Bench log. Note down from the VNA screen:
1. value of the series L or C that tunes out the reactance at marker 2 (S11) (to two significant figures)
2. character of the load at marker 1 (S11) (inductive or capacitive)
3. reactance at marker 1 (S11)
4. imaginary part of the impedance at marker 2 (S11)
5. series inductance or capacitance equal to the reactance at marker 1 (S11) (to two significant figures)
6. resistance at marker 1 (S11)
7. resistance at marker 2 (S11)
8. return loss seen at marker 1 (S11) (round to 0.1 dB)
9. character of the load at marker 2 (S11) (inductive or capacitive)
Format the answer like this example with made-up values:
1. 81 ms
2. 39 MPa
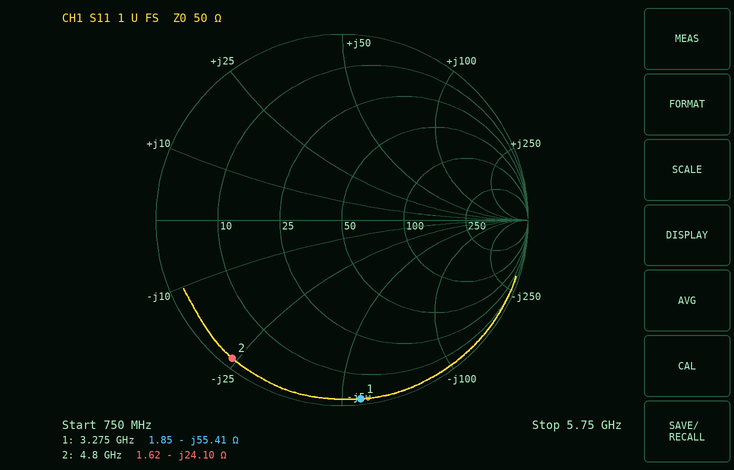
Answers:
1. 800 pH
2. capacitive
3. -55.41 Ω
4. -24.10 Ω
5. 880 fF
6. 1.85 Ω
7. 1.62 Ω
8. 0.3 dB
9. capacitive
